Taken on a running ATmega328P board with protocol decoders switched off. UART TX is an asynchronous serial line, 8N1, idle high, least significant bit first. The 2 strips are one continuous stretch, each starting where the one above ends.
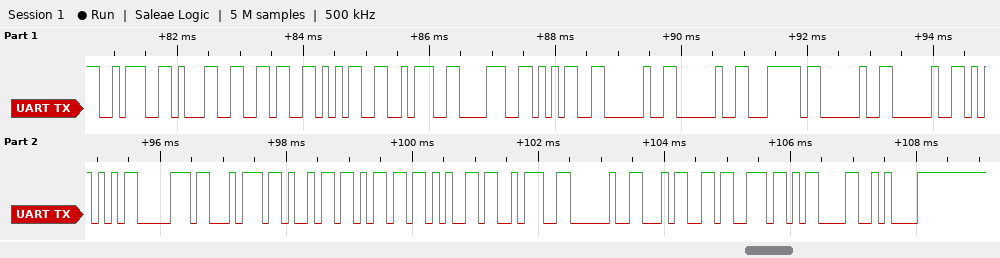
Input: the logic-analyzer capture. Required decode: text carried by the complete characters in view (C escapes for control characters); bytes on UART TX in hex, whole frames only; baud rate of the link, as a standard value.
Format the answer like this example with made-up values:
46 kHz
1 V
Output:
":165:85  |  Uptime: 4s\r\n"
3A 31 36 35 3A 38 35 20 20 7C 20 20 55 70 74 69 6D 65 3A 20 34 73 0D 0A
9600 baud
